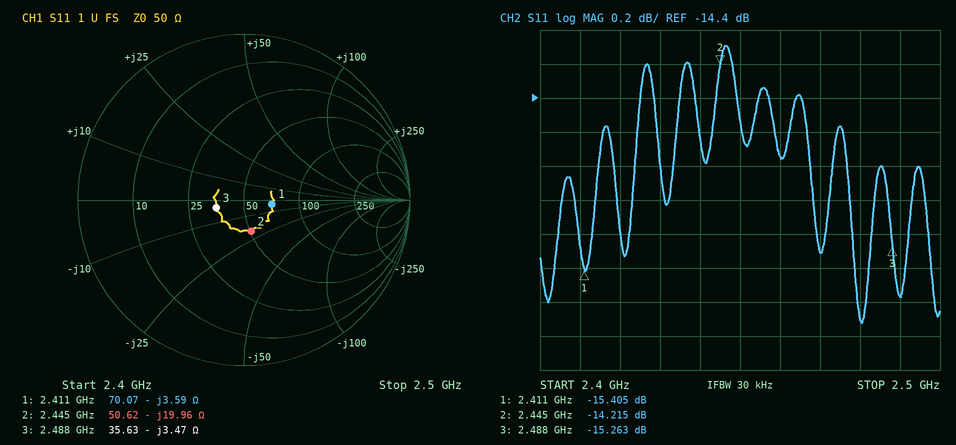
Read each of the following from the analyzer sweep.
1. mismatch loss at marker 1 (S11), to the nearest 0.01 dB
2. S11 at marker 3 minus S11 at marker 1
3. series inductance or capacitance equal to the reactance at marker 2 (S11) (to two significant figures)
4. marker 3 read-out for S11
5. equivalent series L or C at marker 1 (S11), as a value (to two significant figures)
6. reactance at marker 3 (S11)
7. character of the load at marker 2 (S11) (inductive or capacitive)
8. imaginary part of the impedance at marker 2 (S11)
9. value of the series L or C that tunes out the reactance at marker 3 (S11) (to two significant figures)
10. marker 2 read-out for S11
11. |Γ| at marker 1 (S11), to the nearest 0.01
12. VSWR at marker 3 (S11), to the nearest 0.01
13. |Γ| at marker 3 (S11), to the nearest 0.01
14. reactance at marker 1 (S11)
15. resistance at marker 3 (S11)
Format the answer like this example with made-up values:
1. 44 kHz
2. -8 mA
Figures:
1. 0.13 dB
2. 0.142 dB
3. 3.3 pF
4. -15.263 dB
5. 18 pF
6. -3.47 Ω
7. capacitive
8. -19.96 Ω
9. 220 pH
10. -14.215 dB
11. 0.17
12. 1.42
13. 0.17
14. -3.59 Ω
15. 35.63 Ω
